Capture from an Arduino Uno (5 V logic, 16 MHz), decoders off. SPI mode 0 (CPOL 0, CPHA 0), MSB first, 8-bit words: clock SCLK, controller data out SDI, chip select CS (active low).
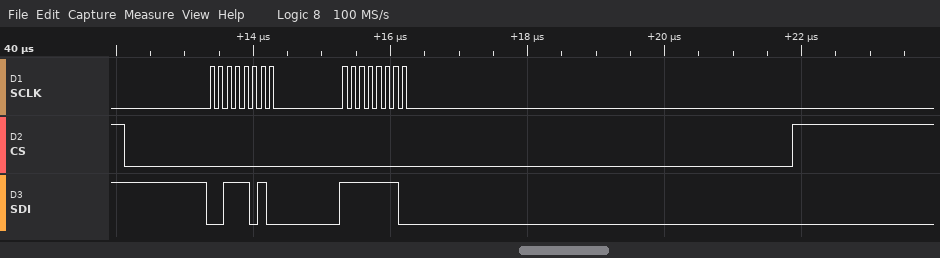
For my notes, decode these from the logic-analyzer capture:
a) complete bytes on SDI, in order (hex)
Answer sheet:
0x3A 0xFE
